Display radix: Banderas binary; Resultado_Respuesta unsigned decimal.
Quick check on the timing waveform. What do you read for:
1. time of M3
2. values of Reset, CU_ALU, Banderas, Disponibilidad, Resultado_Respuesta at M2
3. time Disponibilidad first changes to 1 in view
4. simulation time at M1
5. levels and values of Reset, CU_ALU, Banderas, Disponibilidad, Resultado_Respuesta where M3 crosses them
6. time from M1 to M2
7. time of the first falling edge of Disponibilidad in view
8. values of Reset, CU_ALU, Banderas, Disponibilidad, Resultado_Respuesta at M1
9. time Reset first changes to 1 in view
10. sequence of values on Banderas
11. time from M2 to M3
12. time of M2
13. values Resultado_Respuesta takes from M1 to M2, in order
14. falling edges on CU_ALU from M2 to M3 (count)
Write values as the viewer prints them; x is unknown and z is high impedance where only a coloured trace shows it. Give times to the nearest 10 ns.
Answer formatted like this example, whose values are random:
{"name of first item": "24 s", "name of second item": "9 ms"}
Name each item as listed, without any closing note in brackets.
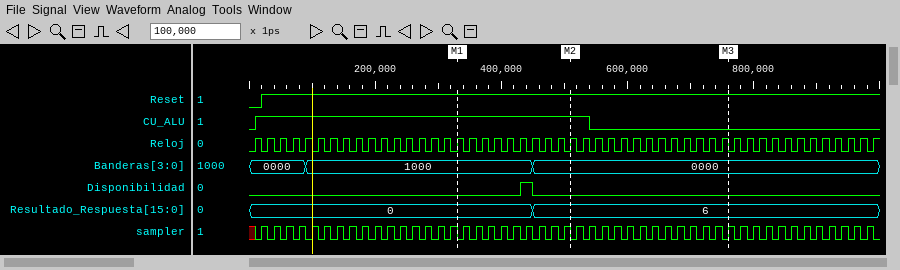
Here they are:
{"time of M3": "760 ns", "values of Reset, CU_ALU, Banderas, Disponibilidad, Resultado_Respuesta at M2": "Reset=1, CU_ALU=1, Banderas=0000, Disponibilidad=0, Resultado_Respuesta=6", "time Disponibilidad first changes to 1 in view": "430 ns", "simulation time at M1": "330 ns", "levels and values of Reset, CU_ALU, Banderas, Disponibilidad, Resultado_Respuesta where M3 crosses them": "Reset=1, CU_ALU=0, Banderas=0000, Disponibilidad=0, Resultado_Respuesta=6", "time from M1 to M2": "180 ns", "time of the first falling edge of Disponibilidad in view": "450 ns", "values of Reset, CU_ALU, Banderas, Disponibilidad, Resultado_Respuesta at M1": "Reset=1, CU_ALU=1, Banderas=1000, Disponibilidad=0, Resultado_Respuesta=0", "time Reset first changes to 1 in view": "20 ns", "sequence of values on Banderas": "0000, 1000, 0000", "time from M2 to M3": "250 ns", "time of M2": "510 ns", "values Resultado_Respuesta takes from M1 to M2, in order": "0, 6", "falling edges on CU_ALU from M2 to M3": "1"}
